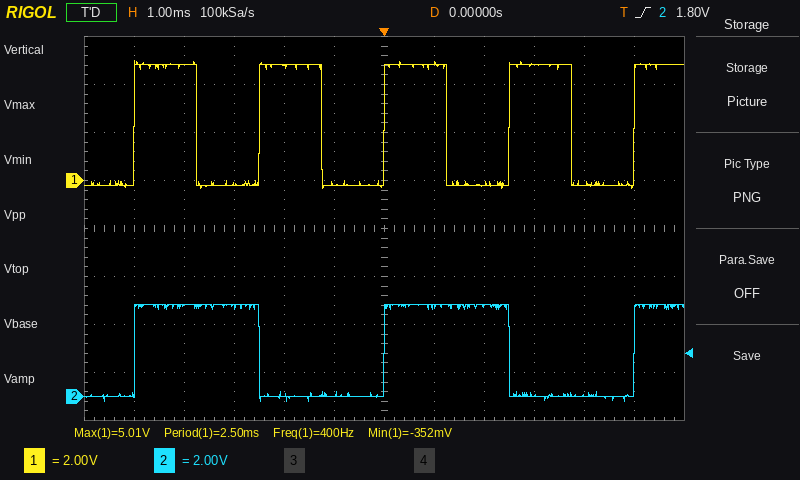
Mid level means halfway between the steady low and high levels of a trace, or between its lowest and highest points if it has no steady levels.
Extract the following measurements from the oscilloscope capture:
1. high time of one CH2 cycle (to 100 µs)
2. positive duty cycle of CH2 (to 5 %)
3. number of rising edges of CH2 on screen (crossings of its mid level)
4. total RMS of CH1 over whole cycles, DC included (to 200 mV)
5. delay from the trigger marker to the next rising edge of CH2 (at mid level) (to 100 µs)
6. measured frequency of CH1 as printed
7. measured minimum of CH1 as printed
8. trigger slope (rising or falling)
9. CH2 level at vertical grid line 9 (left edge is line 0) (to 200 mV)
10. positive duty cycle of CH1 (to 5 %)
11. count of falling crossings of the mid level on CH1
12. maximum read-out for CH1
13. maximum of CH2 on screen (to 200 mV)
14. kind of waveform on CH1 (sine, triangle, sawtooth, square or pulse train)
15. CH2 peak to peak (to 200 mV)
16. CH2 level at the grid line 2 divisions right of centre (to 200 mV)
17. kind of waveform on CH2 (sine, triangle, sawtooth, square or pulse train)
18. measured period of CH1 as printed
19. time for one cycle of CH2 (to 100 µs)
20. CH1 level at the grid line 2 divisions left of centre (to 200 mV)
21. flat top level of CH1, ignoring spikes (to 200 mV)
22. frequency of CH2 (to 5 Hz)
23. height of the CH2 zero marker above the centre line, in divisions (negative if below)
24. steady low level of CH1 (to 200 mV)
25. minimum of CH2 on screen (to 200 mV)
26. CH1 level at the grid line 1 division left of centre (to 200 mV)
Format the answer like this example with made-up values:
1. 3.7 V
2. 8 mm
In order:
1. 2.5 ms
2. 50 %
3. 3
4. 3.4 V
5. 5.0 ms
6. 400 Hz
7. -352 mV
8. rising
9. 0.0 V
10. 50 %
11. 4
12. 5.01 V
13. 3.8 V
14. square
15. 4.0 V
16. 3.8 V
17. square
18. 2.50 ms
19. 5.0 ms
20. 4.8 V
21. 4.8 V
22. 200 Hz
23. -3.5 div
24. -200 mV
25. -200 mV
26. -200 mV
